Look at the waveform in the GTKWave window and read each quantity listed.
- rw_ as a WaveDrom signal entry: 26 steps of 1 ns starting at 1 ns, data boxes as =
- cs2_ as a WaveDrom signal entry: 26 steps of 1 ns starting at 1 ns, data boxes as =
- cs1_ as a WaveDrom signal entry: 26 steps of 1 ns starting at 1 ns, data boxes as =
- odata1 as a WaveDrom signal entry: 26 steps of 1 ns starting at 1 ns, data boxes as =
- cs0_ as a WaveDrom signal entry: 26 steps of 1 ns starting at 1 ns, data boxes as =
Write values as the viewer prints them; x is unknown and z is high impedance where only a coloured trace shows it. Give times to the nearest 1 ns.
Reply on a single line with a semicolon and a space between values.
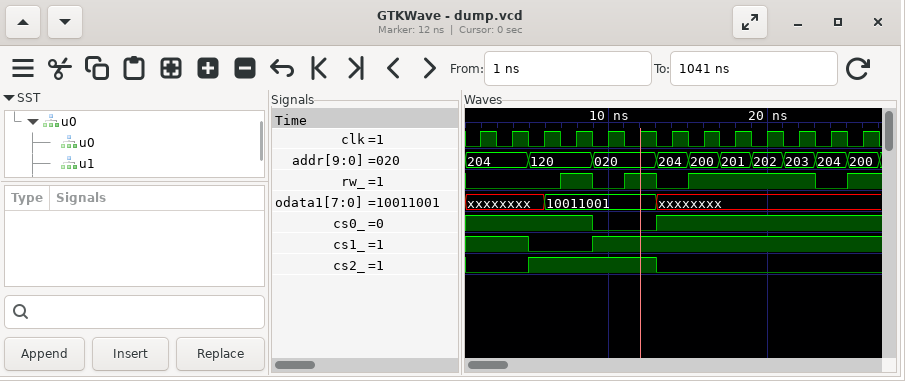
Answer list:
{name: 'rw_', wave: '0.....1.0.1.0.1.......0.1.'}; {name: 'cs2_', wave: '0...1.......0.............'}; {name: 'cs1_', wave: '1...0...1.................'}; {name: 'odata1', wave: 'x....=......x.............', data: '10011001'}; {name: 'cs0_', wave: '1.......0...1.............'}
